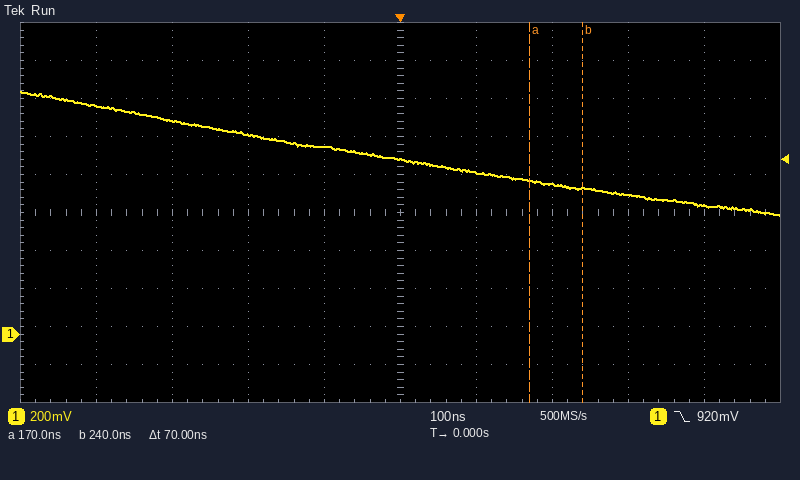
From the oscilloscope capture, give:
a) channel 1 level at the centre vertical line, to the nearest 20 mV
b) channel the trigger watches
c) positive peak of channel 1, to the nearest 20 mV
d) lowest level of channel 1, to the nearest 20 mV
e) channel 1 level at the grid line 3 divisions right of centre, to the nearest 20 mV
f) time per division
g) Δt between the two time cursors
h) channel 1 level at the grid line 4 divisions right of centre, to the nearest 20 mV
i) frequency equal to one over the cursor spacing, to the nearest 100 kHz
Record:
920 mV
channel 1
1.28 V
620 mV
740 mV
100 ns
70 ns
680 mV
14.3 MHz
